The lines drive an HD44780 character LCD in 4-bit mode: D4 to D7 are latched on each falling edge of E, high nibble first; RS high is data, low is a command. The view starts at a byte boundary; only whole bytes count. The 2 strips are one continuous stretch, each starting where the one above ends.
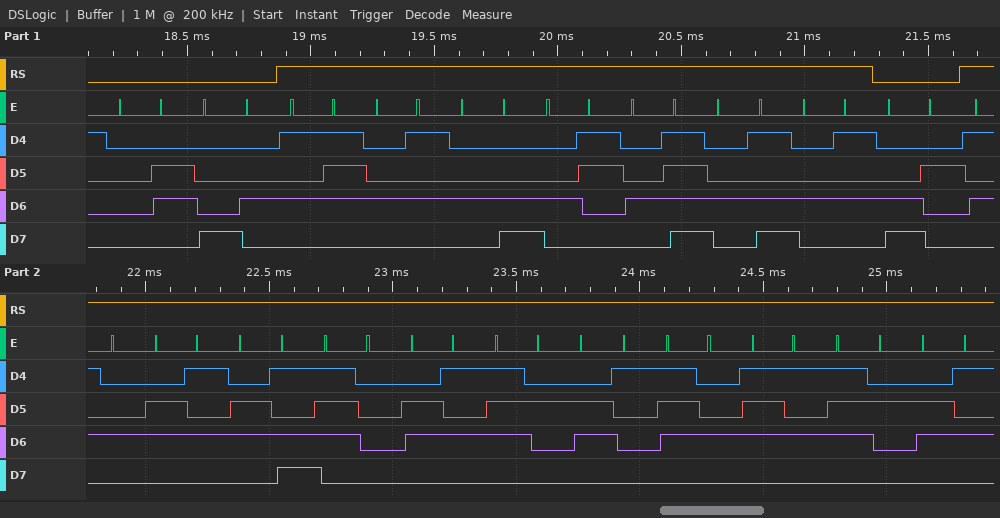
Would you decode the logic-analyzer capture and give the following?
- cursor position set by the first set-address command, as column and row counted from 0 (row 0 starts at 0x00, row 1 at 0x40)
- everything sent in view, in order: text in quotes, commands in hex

column 4, row 0
0x06 0x84 "WELCOME" 0xC2 "Temperature"
